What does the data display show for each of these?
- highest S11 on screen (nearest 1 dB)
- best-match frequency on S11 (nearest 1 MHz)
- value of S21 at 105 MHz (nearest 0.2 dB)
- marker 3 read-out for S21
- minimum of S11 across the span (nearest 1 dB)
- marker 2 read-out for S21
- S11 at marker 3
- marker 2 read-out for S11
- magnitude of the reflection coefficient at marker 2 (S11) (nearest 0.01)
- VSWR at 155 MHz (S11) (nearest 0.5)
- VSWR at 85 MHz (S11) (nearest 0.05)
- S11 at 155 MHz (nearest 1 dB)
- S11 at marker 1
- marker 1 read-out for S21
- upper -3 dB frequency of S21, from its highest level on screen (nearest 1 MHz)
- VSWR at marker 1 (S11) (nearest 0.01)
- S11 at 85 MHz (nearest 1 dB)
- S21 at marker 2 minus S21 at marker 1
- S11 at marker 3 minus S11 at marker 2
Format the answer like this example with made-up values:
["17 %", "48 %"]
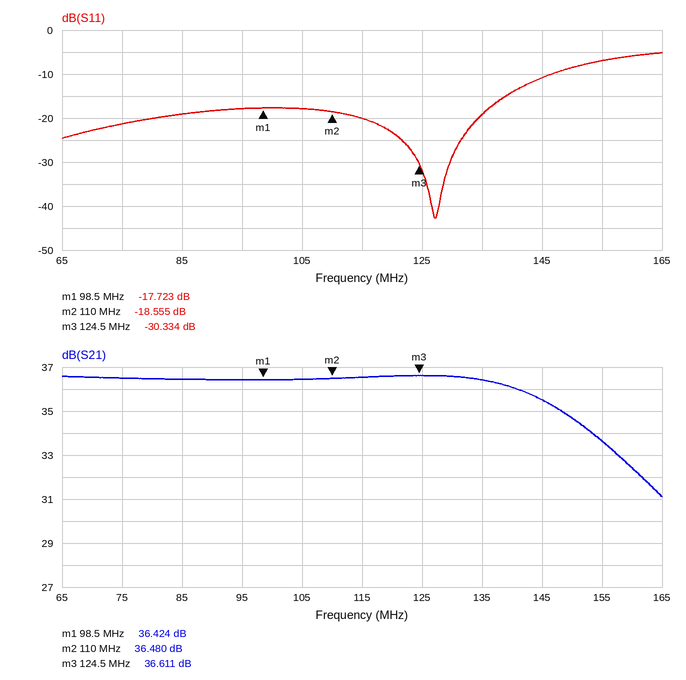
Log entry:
["-5 dB", "127 MHz", "36.4 dB", "36.611 dB", "-43 dB", "36.480 dB", "-30.334 dB", "-18.555 dB", "0.12", "2.5", "1.25", "-7 dB", "-17.723 dB", "36.424 dB", "155 MHz", "1.30", "-19 dB", "0.056 dB", "-11.779 dB"]
